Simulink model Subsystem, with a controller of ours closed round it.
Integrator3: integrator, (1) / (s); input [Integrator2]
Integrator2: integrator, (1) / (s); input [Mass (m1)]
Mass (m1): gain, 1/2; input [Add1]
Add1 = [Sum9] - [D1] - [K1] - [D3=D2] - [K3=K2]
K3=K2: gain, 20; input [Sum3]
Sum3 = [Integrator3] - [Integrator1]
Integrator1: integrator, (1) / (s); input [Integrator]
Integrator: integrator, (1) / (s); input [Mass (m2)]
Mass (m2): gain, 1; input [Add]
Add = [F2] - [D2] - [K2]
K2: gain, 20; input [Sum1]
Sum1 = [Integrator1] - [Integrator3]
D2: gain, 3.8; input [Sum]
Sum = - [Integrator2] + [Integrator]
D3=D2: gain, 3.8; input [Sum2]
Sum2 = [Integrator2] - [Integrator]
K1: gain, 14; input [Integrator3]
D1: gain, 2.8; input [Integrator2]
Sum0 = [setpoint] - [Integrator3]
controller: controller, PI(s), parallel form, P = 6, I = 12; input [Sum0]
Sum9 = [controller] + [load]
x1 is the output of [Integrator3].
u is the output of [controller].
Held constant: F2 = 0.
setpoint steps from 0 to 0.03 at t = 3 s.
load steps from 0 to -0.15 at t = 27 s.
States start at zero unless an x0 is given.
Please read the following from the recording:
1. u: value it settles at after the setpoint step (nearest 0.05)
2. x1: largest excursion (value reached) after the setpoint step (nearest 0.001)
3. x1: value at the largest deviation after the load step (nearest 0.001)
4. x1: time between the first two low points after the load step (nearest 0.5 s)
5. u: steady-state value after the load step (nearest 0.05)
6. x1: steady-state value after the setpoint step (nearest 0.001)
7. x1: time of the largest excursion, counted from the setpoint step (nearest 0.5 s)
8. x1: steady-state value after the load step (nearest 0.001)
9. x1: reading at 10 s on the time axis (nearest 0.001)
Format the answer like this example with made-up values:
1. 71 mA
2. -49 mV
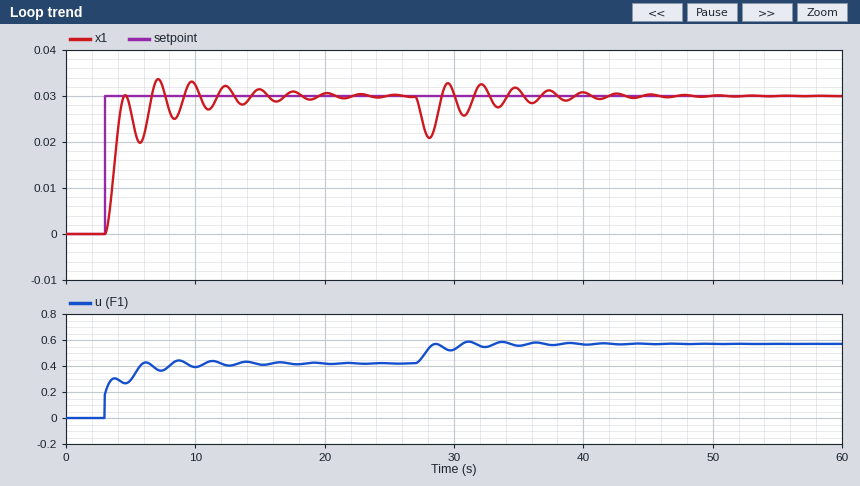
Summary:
1. 0.40
2. 0.034
3. 0.021
4. 2.5 s
5. 0.55
6. 0.030
7. 4.0 s
8. 0.030
9. 0.032
